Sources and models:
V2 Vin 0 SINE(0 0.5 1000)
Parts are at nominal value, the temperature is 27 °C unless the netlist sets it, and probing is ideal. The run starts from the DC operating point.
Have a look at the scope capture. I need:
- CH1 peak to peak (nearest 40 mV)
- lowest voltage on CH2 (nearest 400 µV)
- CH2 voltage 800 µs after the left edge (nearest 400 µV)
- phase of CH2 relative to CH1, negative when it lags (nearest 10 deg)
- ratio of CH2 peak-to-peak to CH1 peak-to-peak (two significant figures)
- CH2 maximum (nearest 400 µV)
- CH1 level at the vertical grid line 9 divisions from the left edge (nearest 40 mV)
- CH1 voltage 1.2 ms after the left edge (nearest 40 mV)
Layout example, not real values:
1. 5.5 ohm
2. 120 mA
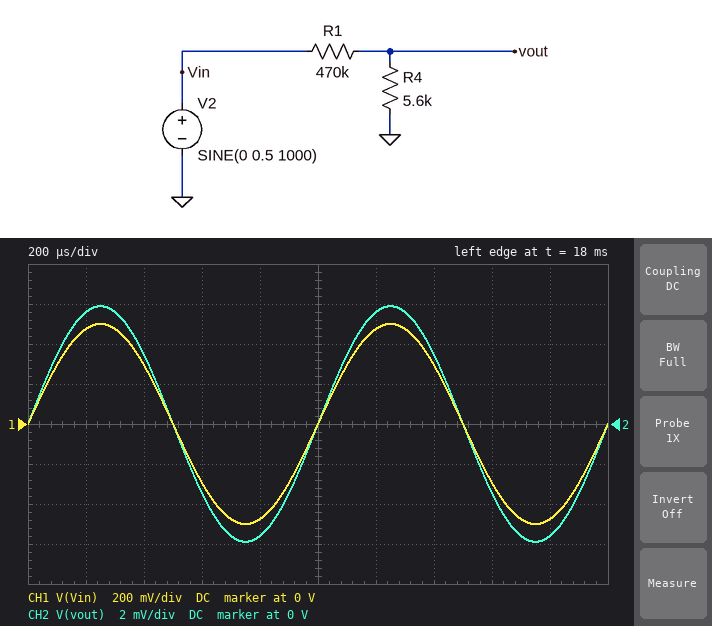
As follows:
1. 1.00 V
2. -6.0 mV
3. -5.6 mV
4. 0 deg
5. 0.012
6. 6.0 mV
7. -480 mV
8. 480 mV
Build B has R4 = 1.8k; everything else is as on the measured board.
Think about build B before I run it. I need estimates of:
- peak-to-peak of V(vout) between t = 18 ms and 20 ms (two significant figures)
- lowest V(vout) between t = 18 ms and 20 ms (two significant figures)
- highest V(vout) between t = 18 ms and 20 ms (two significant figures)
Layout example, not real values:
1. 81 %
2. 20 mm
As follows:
1. 3.8 mV
2. -1.9 mV
3. 1.9 mV
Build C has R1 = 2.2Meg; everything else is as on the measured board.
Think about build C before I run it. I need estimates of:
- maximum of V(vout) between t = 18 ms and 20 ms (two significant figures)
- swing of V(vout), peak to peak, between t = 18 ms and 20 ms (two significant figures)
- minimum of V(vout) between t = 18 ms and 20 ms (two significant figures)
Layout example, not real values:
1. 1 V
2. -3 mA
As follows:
1. 1.3 mV
2. 2.5 mV
3. -1.3 mV
